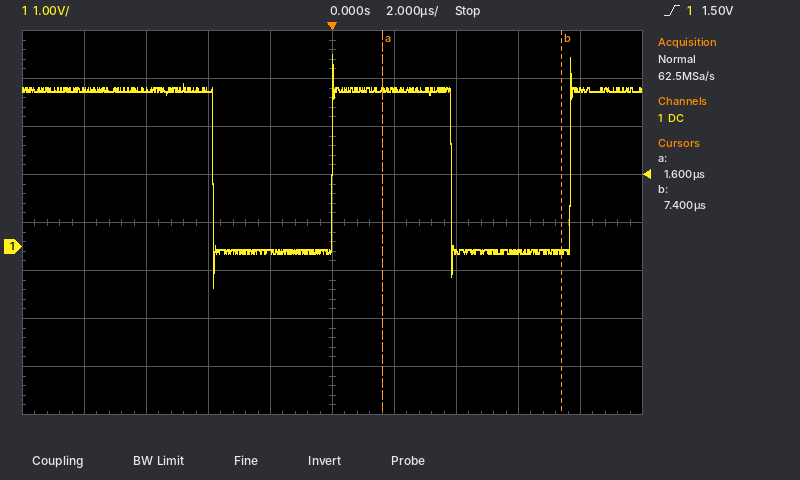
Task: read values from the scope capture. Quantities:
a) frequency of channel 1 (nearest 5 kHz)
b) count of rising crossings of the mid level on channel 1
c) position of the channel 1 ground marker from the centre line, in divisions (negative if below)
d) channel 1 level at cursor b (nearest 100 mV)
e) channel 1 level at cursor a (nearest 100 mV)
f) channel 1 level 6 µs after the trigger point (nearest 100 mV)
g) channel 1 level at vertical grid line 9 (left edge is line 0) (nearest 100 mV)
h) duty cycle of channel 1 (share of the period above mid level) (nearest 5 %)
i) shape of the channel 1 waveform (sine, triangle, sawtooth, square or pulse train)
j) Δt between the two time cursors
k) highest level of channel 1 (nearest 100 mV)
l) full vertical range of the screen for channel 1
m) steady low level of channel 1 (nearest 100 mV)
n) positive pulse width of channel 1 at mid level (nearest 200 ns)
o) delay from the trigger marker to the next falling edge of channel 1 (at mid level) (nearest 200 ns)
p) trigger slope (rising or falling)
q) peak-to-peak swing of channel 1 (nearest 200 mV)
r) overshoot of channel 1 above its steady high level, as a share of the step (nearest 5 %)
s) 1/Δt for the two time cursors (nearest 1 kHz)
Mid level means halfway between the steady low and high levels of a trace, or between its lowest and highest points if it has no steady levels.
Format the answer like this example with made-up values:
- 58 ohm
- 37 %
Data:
- 130 kHz
- 2
- -0.5 div
- -100 mV
- 3.3 V
- -100 mV
- 3.3 V
- 50 %
- square
- 5.8 µs
- 4.0 V
- 8 V
- -100 mV
- 3.8 µs
- 3.8 µs
- rising
- 4.8 V
- 20 %
- 172 kHz
